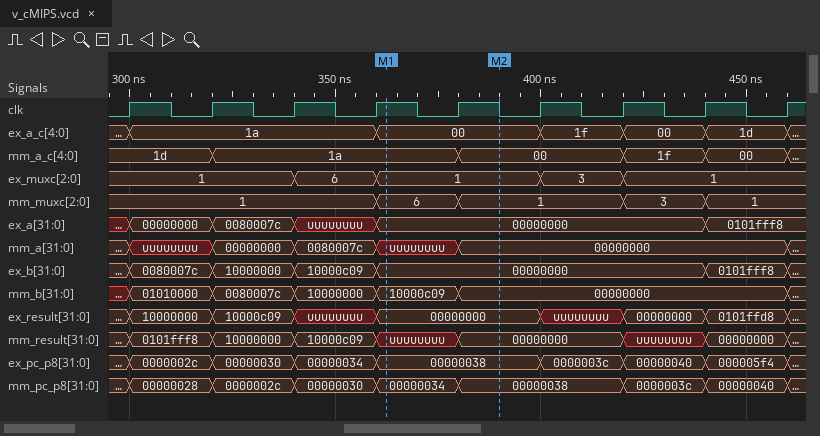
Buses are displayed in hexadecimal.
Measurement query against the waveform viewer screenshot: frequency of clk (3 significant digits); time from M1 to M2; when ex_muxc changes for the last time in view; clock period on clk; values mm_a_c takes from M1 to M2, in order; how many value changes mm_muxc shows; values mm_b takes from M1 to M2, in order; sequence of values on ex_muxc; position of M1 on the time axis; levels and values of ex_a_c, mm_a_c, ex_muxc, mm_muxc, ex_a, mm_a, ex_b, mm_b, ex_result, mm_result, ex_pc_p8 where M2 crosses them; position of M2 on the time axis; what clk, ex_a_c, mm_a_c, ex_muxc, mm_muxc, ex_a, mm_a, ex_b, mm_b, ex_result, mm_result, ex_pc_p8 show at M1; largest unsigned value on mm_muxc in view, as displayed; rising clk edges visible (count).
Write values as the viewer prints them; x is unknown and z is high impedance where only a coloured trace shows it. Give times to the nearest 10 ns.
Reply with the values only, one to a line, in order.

50.0 MHz
30 ns
420 ns
20 ns
1a, 00
4
10000c09, 00000000
1, 6, 1, 3, 1
360 ns
ex_a_c=00, mm_a_c=00, ex_muxc=1, mm_muxc=1, ex_a=00000000, mm_a=00000000, ex_b=00000000, mm_b=00000000, ex_result=00000000, mm_result=00000000, ex_pc_p8=00000038
390 ns
clk=1, ex_a_c=00, mm_a_c=1a, ex_muxc=1, mm_muxc=6, ex_a=00000000, mm_a=uuuuuuuu, ex_b=00000000, mm_b=10000c09, ex_result=00000000, mm_result=uuuuuuuu, ex_pc_p8=00000038
6
9
